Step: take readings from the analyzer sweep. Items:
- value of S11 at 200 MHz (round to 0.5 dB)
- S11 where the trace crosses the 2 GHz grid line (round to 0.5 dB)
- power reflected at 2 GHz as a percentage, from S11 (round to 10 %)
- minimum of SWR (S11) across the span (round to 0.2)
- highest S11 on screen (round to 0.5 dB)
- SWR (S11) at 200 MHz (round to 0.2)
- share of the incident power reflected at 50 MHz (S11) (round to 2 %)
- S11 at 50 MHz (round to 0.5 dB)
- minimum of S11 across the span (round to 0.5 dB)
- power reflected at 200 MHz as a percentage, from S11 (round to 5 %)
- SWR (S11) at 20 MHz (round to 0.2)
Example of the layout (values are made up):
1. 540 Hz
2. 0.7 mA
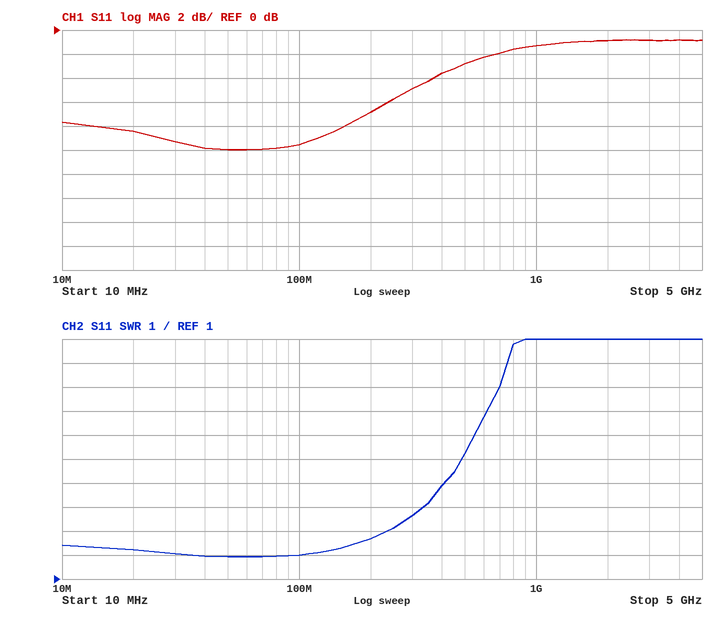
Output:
1. -7.0 dB
2. -1.0 dB
3. 80 %
4. 2.0
5. -1.0 dB
6. 2.6
7. 10 %
8. -10.0 dB
9. -10.0 dB
10. 20 %
11. 2.2
